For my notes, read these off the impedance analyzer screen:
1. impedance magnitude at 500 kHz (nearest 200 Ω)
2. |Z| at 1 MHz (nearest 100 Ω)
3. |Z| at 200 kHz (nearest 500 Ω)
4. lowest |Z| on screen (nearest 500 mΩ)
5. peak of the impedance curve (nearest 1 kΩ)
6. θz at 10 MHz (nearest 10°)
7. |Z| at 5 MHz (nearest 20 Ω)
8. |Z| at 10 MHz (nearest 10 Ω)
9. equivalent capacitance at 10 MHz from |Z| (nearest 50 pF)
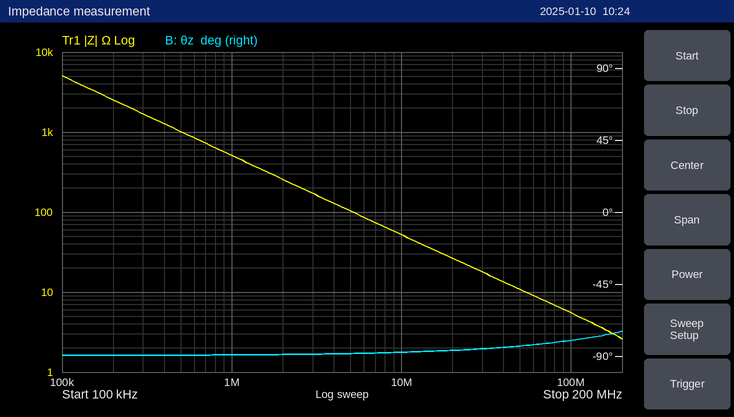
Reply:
1.0 kΩ
500 Ω
2.5 kΩ
2.5 Ω
5 kΩ
-90°
100 Ω
50 Ω
300 pF
